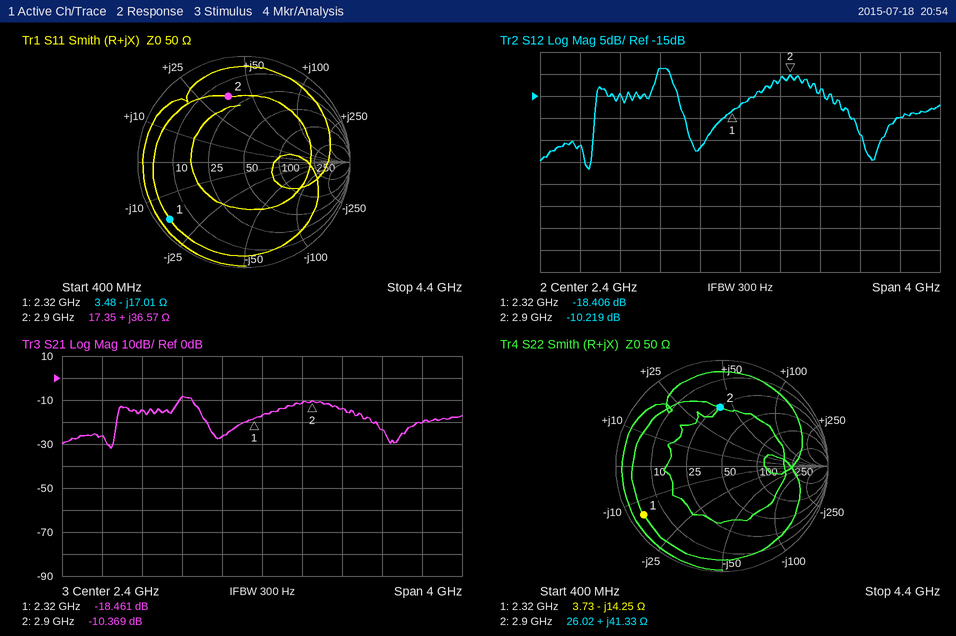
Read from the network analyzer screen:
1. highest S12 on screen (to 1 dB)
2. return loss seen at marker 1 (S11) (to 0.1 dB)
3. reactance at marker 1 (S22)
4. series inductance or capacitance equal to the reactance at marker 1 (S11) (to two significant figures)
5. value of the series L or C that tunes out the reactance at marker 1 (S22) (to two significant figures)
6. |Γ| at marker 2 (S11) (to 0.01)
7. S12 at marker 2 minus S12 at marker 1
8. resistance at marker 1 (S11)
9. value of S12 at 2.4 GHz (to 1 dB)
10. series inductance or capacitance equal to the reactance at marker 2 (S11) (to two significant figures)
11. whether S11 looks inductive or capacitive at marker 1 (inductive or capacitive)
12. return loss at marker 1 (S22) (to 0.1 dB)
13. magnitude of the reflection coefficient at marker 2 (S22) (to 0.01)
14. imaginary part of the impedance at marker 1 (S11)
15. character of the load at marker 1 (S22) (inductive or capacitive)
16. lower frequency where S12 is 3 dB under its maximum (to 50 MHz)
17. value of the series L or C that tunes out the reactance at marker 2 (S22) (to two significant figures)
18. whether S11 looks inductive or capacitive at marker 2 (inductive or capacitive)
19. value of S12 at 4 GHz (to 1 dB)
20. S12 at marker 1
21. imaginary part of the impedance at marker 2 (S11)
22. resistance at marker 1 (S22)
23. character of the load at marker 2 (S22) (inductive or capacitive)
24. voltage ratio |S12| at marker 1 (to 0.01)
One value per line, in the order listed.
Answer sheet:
-9 dB
1.1 dB
-14.25 Ω
4.0 pF
980 pH
0.64
8.187 dB
3.48 Ω
-17 dB
2.0 nH
capacitive
1.2 dB
0.55
-17.01 Ω
capacitive
1.55 GHz
1.3 pF
inductive
-20 dB
-18.406 dB
+36.57 Ω
3.73 Ω
inductive
0.12
